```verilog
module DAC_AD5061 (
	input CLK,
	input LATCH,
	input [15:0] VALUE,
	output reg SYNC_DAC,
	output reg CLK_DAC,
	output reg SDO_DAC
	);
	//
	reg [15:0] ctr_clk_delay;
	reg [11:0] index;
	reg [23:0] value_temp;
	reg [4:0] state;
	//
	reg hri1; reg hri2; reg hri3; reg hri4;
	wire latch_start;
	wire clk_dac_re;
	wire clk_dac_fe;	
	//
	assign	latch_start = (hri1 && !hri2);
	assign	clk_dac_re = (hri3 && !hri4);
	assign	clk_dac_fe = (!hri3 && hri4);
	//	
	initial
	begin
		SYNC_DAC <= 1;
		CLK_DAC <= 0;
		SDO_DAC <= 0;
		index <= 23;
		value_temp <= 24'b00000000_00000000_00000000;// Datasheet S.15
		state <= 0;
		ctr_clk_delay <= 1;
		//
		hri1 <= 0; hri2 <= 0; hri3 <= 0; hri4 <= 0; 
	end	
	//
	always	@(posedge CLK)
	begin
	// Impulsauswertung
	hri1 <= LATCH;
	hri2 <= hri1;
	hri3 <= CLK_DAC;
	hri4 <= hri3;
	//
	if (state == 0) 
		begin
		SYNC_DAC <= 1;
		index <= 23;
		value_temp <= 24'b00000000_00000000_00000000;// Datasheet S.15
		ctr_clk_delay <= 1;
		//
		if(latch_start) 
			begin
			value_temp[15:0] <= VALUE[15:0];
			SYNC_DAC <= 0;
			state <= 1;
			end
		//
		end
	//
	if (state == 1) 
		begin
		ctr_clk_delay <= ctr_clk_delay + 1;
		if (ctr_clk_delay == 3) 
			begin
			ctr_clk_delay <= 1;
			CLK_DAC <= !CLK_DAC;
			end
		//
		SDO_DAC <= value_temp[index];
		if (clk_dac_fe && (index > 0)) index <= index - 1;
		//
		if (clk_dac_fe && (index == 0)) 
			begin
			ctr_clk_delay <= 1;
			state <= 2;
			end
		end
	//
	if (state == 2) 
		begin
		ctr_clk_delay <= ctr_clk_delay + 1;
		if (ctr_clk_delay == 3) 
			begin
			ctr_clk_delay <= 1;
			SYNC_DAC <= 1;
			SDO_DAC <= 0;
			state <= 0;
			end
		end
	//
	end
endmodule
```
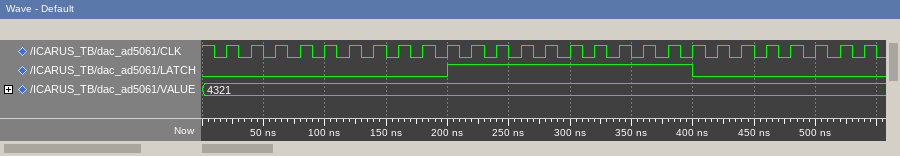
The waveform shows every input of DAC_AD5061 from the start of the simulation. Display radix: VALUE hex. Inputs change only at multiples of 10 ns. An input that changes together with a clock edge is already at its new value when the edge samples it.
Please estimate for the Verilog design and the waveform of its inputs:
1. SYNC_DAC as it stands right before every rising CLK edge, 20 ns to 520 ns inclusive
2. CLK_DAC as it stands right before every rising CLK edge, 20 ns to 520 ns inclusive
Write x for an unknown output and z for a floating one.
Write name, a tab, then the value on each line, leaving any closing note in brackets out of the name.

SYNC_DAC as it stands right before every rising CLK edge, 20 ns to 520 ns inclusive	1 1 1 1 1 1 1 1 1 1 1 0 0 0 0 0 0 0 0 0 0 0 0 0 0 0
CLK_DAC as it stands right before every rising CLK edge, 20 ns to 520 ns inclusive	0 0 0 0 0 0 0 0 0 0 0 0 0 0 1 1 1 0 0 0 1 1 1 0 0 0
